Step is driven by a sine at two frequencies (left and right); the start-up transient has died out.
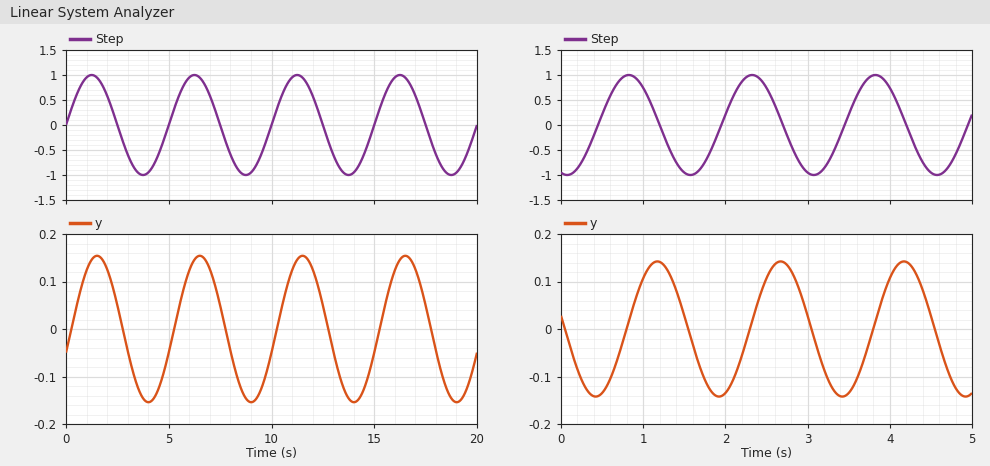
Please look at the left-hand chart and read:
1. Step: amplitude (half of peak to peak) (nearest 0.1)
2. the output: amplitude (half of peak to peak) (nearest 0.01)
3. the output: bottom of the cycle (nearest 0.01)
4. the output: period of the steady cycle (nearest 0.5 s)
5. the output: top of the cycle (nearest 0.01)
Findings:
1.0
0.15
-0.15
5.0 s
0.15
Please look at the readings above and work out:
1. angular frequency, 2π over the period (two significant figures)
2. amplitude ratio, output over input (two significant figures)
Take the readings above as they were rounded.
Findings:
1.3 rad/s
0.15
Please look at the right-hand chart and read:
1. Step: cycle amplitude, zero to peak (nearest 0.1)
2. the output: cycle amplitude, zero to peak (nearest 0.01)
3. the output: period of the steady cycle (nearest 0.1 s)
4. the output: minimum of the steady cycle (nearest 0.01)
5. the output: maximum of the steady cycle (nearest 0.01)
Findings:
1.0
0.14
1.5 s
-0.14
0.14
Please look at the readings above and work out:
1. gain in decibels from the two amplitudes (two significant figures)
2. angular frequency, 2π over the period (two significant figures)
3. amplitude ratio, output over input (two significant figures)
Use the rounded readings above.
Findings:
-17 dB
4.2 rad/s
0.14
